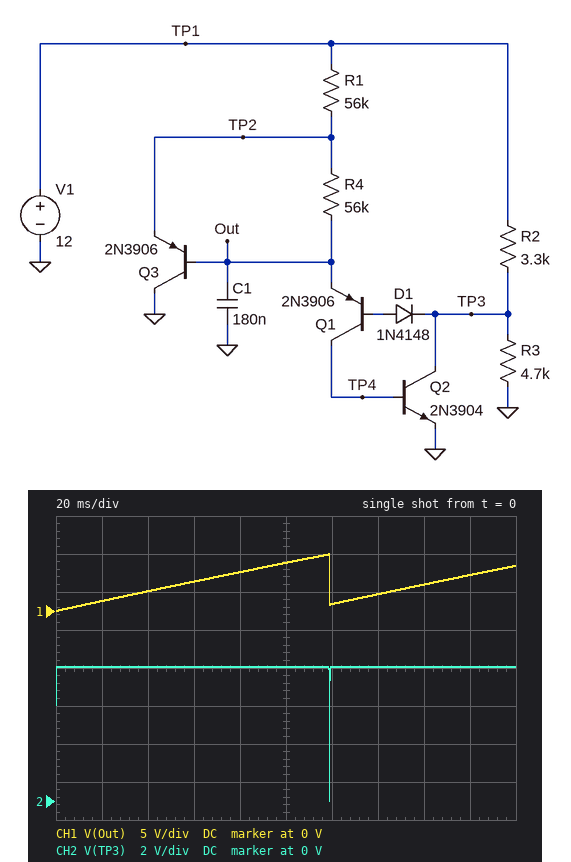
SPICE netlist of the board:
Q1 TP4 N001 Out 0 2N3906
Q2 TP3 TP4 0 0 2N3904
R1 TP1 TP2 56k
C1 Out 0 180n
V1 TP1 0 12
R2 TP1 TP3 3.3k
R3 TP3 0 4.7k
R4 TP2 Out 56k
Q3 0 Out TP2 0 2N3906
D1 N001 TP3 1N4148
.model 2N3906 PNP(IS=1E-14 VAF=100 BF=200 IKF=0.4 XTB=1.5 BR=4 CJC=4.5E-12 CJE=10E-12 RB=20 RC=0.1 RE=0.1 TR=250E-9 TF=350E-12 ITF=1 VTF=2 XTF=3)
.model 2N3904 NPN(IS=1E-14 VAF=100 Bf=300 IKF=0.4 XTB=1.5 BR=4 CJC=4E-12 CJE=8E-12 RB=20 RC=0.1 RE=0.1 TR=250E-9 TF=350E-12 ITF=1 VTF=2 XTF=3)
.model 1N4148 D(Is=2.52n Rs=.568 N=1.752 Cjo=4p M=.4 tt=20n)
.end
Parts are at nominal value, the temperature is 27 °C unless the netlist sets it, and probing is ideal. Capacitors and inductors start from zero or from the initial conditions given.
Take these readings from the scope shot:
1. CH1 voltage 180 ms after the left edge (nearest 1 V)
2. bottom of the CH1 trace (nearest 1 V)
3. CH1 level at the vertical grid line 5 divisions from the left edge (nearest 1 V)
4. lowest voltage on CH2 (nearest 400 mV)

5 V
0 V
6 V
0 V
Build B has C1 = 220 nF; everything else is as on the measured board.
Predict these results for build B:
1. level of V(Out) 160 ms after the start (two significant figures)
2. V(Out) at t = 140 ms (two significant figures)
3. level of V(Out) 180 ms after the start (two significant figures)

1.6 V
7.2 V
2.7 V
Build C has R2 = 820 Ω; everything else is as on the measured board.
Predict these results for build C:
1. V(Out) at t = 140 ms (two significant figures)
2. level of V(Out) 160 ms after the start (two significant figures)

8.7 V
9.8 V
